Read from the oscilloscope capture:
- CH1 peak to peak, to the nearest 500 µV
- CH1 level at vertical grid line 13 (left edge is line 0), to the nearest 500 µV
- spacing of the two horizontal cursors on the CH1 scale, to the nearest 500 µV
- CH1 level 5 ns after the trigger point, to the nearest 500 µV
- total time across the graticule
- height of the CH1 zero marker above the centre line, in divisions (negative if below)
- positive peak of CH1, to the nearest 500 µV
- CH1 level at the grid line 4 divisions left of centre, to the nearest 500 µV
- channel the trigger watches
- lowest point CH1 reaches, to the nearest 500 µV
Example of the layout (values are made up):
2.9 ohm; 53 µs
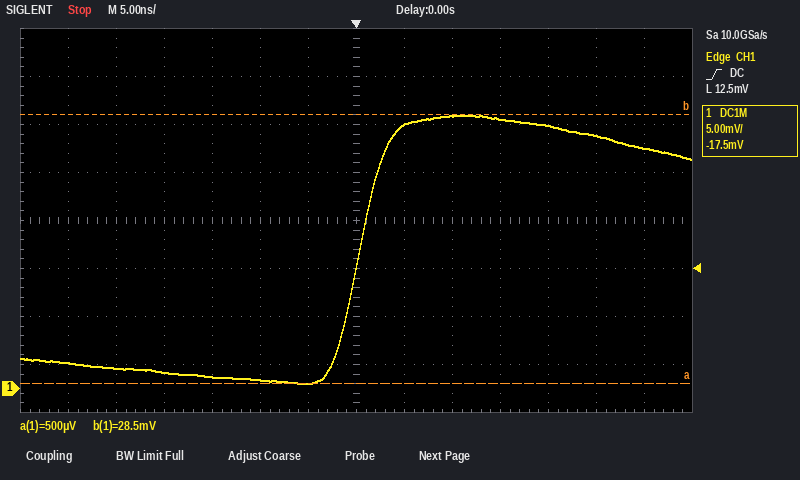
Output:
28.0 mV; 25.0 mV; 28.0 mV; 27.5 mV; 70 ns; -3.5 div; 28.5 mV; 1.5 mV; CH1; 500 µV
